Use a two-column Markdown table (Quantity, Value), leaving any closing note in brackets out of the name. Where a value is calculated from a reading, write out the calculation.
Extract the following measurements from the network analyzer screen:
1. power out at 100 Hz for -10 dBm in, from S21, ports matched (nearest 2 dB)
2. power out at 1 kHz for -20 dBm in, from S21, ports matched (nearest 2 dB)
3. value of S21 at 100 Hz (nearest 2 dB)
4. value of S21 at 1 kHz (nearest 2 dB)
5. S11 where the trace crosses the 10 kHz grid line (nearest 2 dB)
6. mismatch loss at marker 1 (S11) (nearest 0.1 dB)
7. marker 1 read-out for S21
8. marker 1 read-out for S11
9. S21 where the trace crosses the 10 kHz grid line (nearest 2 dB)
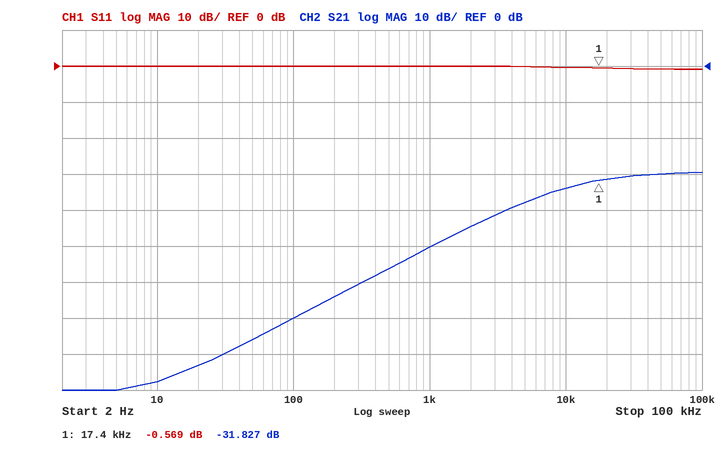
| Quantity | Value |
|---|---|
| power out at 100 Hz for -10 dBm in, from S21, ports matched | -10 dBm + (-70 dB) = -80 dBm |
| power out at 1 kHz for -20 dBm in, from S21, ports matched | -20 dBm + (-50 dB) = -70 dBm |
| value of S21 at 100 Hz | -70 dB |
| value of S21 at 1 kHz | -50 dB |
| S11 where the trace crosses the 10 kHz grid line | 0 dB |
| mismatch loss at marker 1 (S11) | −10 log10(1 − 10^(-0.569/10)) ≈ 9.1 dB |
| marker 1 read-out for S21 | -31.827 dB |
| marker 1 read-out for S11 | -0.569 dB |
| S21 where the trace crosses the 10 kHz grid line | -34 dB |
